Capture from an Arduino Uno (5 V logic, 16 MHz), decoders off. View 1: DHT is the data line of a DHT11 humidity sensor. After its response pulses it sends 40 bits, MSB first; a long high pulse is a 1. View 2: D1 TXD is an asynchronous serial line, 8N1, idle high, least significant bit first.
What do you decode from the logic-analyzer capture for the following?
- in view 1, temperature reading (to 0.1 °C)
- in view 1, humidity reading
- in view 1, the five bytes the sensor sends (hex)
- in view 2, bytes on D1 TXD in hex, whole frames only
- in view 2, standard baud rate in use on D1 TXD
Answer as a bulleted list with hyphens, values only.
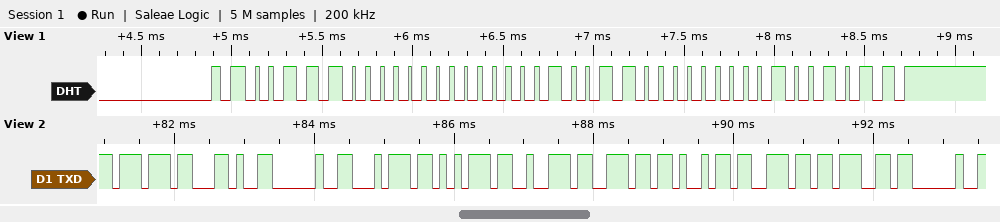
- 19.0 °C
- 56 %
- 38 00 13 00 4B
- 77 2C 20 74 75 72 6E 69 6E 67 20
- 9600 baud
